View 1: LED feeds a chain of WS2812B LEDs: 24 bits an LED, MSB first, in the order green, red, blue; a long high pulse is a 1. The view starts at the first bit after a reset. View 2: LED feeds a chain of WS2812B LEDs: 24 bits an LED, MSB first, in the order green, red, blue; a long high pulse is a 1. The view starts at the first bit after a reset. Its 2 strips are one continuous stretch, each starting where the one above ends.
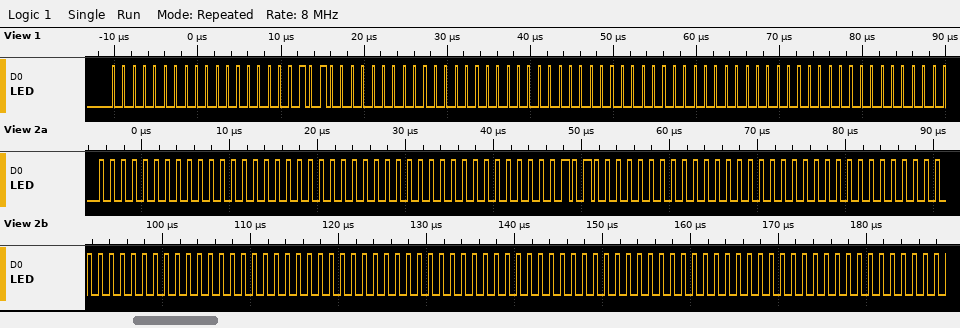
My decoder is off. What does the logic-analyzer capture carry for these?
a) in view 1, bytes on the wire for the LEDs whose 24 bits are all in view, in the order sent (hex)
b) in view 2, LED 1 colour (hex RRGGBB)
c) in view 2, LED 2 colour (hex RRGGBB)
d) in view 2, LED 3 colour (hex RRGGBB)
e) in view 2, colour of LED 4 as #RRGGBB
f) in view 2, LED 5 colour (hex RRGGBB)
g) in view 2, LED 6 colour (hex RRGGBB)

00 00 28 00 00 00 00 00 00
#000000
#000028
#000000
#000000
#000000
#000000
